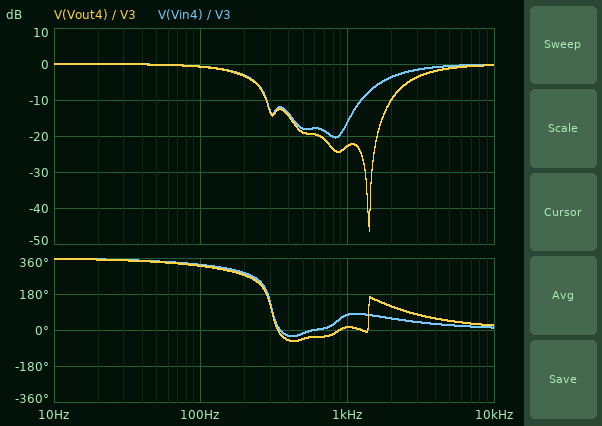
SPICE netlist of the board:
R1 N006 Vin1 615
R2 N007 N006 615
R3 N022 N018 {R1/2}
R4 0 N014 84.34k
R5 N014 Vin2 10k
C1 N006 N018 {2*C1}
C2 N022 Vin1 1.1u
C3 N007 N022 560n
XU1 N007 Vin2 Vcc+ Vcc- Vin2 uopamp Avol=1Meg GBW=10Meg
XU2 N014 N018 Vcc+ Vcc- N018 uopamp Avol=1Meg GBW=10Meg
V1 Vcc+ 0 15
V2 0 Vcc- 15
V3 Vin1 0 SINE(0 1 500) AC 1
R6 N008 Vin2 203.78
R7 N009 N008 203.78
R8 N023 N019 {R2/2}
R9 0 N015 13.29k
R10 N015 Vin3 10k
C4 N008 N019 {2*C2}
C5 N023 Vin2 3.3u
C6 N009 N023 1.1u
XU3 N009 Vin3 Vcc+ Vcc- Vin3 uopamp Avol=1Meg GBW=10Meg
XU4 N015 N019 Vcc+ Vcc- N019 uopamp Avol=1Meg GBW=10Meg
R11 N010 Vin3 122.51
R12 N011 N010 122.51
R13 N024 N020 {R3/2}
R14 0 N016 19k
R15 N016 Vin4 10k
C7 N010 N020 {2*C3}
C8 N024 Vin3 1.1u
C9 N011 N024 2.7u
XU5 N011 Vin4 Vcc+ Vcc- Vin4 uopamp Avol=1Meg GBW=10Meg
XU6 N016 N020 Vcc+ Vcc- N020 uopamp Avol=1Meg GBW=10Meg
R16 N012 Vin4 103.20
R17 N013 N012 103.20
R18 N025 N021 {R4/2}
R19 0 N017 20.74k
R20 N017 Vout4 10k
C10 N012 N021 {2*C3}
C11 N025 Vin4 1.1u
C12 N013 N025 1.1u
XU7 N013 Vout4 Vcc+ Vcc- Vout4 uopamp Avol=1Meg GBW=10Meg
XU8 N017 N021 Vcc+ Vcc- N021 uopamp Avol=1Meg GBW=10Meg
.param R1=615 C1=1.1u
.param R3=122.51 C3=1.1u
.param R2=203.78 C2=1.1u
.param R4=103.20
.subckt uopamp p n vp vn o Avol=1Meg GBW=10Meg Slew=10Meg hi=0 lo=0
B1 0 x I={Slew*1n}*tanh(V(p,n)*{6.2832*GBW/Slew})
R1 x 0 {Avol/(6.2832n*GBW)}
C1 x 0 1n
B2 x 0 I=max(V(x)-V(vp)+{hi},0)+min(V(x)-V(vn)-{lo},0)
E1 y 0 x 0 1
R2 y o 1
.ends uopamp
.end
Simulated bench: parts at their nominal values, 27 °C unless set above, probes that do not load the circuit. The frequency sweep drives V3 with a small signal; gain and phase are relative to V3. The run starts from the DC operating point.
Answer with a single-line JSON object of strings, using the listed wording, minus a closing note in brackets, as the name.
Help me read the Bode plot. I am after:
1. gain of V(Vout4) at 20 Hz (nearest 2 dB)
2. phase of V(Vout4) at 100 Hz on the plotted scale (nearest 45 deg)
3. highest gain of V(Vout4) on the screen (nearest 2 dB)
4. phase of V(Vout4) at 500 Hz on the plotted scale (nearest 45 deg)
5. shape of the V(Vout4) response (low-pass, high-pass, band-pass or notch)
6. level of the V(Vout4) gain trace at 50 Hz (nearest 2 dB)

{"gain of V(Vout4) at 20 Hz": "0 dB", "phase of V(Vout4) at 100 Hz on the plotted scale": "315 deg", "highest gain of V(Vout4) on the screen": "0 dB", "phase of V(Vout4) at 500 Hz on the plotted scale": "-45 deg", "shape of the V(Vout4) response": "notch", "level of the V(Vout4) gain trace at 50 Hz": "0 dB"}
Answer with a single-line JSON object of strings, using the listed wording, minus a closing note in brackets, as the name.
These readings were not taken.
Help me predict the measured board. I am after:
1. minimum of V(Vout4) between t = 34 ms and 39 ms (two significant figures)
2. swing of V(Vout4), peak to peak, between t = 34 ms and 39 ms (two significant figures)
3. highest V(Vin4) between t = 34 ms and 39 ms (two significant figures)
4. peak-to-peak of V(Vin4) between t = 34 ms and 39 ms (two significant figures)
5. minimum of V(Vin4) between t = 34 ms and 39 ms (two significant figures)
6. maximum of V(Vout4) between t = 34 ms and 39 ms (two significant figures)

{"minimum of V(Vout4) between t = 34 ms and 39 ms": "-110 mV", "swing of V(Vout4), peak to peak, between t = 34 ms and 39 ms": "220 mV", "highest V(Vin4) between t = 34 ms and 39 ms": "130 mV", "peak-to-peak of V(Vin4) between t = 34 ms and 39 ms": "250 mV", "minimum of V(Vin4) between t = 34 ms and 39 ms": "-130 mV", "maximum of V(Vout4) between t = 34 ms and 39 ms": "110 mV"}
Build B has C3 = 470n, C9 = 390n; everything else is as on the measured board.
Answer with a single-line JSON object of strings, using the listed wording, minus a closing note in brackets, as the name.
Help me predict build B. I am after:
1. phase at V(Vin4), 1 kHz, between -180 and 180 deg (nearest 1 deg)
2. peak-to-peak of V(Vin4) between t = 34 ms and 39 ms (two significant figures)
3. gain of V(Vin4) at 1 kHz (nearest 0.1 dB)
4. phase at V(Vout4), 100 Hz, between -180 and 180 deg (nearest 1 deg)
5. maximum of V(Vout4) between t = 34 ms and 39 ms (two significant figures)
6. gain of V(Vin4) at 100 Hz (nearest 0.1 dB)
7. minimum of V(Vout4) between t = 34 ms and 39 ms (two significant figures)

{"phase at V(Vin4), 1 kHz, between -180 and 180 deg": "-13 deg", "peak-to-peak of V(Vin4) between t = 34 ms and 39 ms": "470 mV", "gain of V(Vin4) at 1 kHz": "-6.1 dB", "phase at V(Vout4), 100 Hz, between -180 and 180 deg": "-32 deg", "maximum of V(Vout4) between t = 34 ms and 39 ms": "210 mV", "gain of V(Vin4) at 100 Hz": "-0.5 dB", "minimum of V(Vout4) between t = 34 ms and 39 ms": "-210 mV"}
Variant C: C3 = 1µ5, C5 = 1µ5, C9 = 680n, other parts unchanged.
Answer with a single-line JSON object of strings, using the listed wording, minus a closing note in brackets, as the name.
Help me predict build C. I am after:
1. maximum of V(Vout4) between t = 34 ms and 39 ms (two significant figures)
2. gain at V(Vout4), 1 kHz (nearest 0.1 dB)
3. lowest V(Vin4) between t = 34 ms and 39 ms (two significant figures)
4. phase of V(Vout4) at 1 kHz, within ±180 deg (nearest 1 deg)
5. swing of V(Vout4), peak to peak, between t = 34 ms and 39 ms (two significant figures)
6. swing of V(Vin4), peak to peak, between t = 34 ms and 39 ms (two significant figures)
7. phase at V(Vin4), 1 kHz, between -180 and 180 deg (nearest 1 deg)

{"maximum of V(Vout4) between t = 34 ms and 39 ms": "220 mV", "gain at V(Vout4), 1 kHz": "-18.5 dB", "lowest V(Vin4) between t = 34 ms and 39 ms": "-250 mV", "phase of V(Vout4) at 1 kHz, within ±180 deg": "-70 deg", "swing of V(Vout4), peak to peak, between t = 34 ms and 39 ms": "440 mV", "swing of V(Vin4), peak to peak, between t = 34 ms and 39 ms": "500 mV", "phase at V(Vin4), 1 kHz, between -180 and 180 deg": "-8 deg"}
